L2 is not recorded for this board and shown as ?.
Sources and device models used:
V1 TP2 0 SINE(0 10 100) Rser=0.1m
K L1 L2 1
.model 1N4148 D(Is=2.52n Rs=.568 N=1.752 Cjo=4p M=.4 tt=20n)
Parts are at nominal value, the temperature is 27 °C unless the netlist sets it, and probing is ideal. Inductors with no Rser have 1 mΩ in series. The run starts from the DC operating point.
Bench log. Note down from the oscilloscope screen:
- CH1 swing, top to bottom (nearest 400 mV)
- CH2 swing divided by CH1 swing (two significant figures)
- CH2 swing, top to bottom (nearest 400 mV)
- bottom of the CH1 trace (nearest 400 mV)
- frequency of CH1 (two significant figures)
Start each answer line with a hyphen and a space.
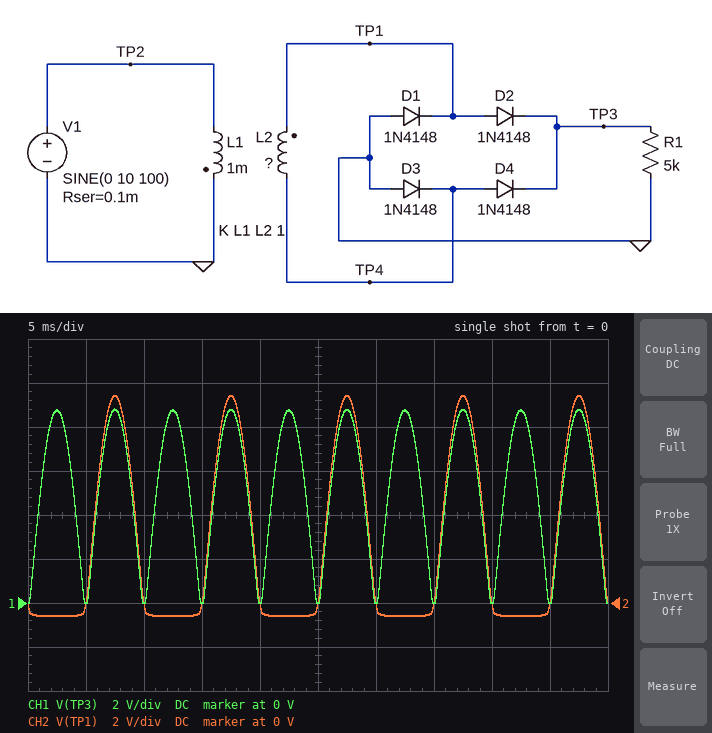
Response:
- 8.8 V
- 1.1
- 10.0 V
- 0 V
- 200 Hz
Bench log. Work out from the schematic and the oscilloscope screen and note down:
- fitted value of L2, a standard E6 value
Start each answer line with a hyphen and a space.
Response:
- 1 mH
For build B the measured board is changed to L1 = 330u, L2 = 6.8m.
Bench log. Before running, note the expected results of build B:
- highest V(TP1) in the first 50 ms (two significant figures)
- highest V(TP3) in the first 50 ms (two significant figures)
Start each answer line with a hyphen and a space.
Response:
- 45 V
- 44 V
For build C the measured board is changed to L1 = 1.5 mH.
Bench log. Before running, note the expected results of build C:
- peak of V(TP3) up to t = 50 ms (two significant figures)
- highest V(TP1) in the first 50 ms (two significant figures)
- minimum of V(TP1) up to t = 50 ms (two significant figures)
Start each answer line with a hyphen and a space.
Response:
- 7.0 V
- 7.6 V
- -600 mV
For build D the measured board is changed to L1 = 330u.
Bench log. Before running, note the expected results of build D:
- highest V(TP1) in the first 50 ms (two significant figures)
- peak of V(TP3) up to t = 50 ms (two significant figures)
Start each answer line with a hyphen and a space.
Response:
- 17 V
- 16 V
